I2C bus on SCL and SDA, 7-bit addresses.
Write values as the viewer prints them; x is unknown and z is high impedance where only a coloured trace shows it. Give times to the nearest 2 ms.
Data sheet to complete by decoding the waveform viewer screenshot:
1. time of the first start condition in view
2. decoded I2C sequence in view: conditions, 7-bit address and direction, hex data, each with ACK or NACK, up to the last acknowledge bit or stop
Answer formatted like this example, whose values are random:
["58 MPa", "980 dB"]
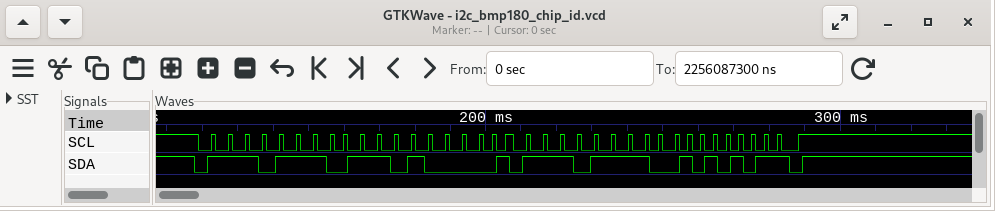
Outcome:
["118 ms", "start, address 77 write ACK, D0 ACK, repeated start, address 77 read ACK, 55 NACK, stop"]
